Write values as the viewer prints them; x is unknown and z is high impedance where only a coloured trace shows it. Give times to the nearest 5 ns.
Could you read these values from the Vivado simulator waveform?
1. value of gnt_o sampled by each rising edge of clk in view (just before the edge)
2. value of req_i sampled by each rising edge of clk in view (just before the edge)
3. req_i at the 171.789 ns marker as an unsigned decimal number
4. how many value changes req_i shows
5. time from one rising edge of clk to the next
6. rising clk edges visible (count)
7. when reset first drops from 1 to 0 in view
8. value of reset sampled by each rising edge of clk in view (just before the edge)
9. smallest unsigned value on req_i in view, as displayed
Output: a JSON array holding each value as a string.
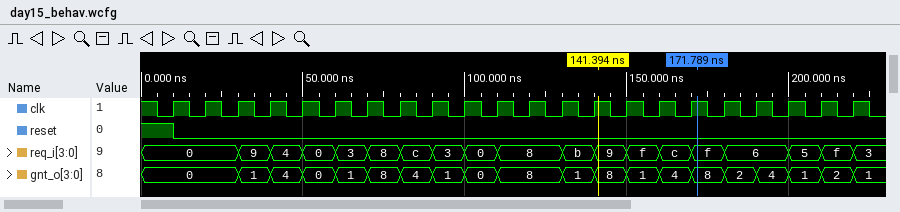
["0, 0, 0, 1, 4, 0, 1, 8, 4, 1, 0, 8, 8, 1, 8, 1, 4, 8, 2, 4, 1, 2", "0, 0, 0, 9, 4, 0, 3, 8, c, 3, 0, 8, 8, b, 9, f, c, f, 6, 6, 5, f", "15", "18", "10 ns", "22", "10 ns", "1 0 0 0 0 0 0 0 0 0 0 0 0 0 0 0 0 0 0 0 0 0", "0"]
